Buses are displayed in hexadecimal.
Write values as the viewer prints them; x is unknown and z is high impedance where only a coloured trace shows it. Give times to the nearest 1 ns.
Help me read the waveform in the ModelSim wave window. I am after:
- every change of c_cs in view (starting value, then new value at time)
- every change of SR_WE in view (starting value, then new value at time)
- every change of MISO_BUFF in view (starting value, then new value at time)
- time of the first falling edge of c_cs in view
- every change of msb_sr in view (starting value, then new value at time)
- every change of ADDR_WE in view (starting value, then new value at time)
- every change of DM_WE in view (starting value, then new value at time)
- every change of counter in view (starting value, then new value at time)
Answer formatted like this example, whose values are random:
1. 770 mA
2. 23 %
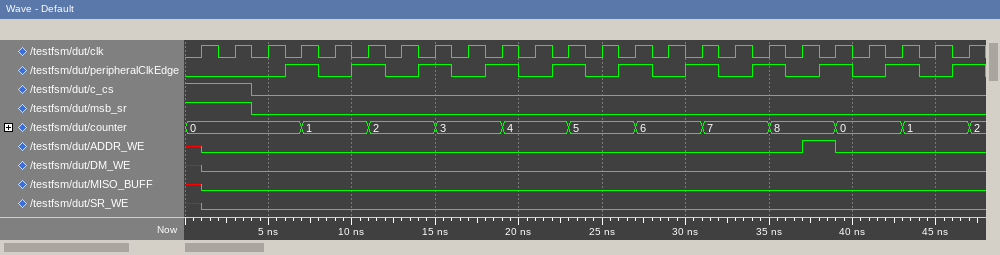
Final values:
1. 1, 0 at 4 ns
2. x, 0 at 1 ns
3. x, 0 at 1 ns
4. 4 ns
5. 1, 0 at 4 ns
6. x, 0 at 1 ns, 1 at 37 ns, 0 at 39 ns
7. x, 0 at 1 ns
8. 0, 1 at 7 ns, 2 at 11 ns, 3 at 15 ns, 4 at 19 ns, 5 at 23 ns, 6 at 27 ns, 7 at 31 ns, 8 at 35 ns, 0 at 39 ns, 1 at 43 ns, 2 at 47 ns
